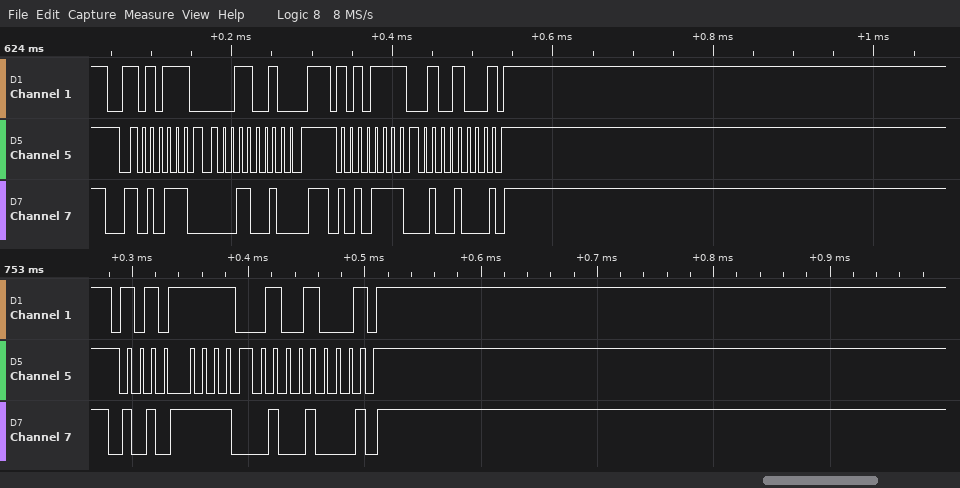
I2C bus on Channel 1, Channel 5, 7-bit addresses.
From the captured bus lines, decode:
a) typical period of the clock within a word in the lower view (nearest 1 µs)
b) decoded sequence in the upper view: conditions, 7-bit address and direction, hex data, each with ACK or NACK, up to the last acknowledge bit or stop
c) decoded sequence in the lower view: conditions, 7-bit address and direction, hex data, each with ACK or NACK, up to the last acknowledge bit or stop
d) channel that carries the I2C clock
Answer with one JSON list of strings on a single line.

["11 µs", "start, address 57 write ACK, 32 ACK, stop, start, address 57 read ACK, 48 NACK, stop", "start, address 57 read ACK, 48 NACK, stop", "Channel 5"]
